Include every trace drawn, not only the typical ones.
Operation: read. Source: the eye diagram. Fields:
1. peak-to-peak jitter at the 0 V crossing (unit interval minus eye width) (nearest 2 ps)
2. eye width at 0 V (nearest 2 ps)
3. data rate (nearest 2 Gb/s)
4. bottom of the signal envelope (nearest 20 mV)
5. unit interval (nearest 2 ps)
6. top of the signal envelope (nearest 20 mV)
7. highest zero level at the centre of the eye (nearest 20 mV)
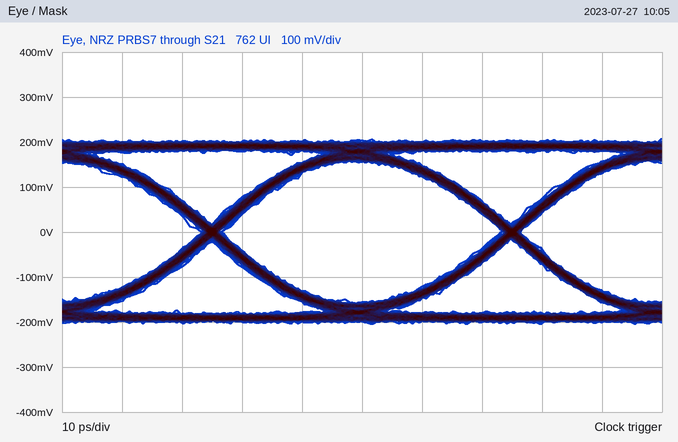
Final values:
4 ps
46 ps
20 Gb/s
-200 mV
50 ps
200 mV
-160 mV
